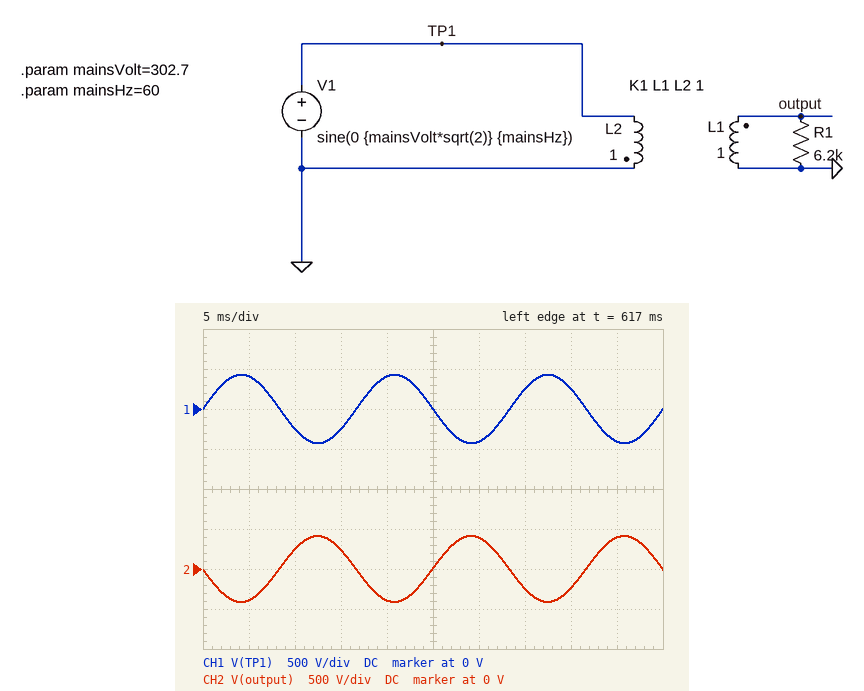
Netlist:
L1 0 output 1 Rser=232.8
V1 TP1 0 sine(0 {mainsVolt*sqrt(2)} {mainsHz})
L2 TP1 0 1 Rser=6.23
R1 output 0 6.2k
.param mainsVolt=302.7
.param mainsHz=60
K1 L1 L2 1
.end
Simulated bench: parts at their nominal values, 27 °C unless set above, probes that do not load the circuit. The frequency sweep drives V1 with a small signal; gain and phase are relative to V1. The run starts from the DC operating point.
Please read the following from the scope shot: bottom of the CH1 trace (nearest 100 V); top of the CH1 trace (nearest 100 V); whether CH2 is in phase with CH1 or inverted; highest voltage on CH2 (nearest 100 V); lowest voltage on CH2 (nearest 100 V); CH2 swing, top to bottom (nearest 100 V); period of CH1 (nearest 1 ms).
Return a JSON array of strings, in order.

["-400 V", "400 V", "inverted", "400 V", "-400 V", "800 V", "17 ms"]
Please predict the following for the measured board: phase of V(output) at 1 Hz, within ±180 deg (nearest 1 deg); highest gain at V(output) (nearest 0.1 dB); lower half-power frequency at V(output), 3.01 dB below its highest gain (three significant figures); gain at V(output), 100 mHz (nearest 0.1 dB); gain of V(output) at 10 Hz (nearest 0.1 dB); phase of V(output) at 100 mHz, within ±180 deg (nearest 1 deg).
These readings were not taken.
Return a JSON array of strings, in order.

["-135 deg", "-0.3 dB", "991 mHz", "-20.3 dB", "-0.4 dB", "-96 deg"]
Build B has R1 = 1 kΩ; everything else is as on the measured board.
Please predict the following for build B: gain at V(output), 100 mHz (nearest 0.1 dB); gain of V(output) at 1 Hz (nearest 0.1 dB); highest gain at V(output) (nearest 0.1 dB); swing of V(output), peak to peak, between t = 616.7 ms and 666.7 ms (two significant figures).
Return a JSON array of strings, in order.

["-21.8 dB", "-4.8 dB", "-1.9 dB", "690 V"]
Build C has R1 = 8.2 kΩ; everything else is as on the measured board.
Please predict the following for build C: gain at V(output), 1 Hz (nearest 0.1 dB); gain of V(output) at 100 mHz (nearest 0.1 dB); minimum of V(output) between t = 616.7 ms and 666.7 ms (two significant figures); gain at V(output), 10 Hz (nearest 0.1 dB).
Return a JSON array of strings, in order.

["-3.2 dB", "-20.2 dB", "-420 V", "-0.3 dB"]
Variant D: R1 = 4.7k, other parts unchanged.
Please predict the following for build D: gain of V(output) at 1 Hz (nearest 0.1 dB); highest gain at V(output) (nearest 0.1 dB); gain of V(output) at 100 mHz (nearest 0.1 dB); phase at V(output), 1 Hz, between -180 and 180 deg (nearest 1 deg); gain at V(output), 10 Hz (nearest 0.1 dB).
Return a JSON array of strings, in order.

["-3.4 dB", "-0.4 dB", "-20.4 dB", "-135 deg", "-0.5 dB"]
